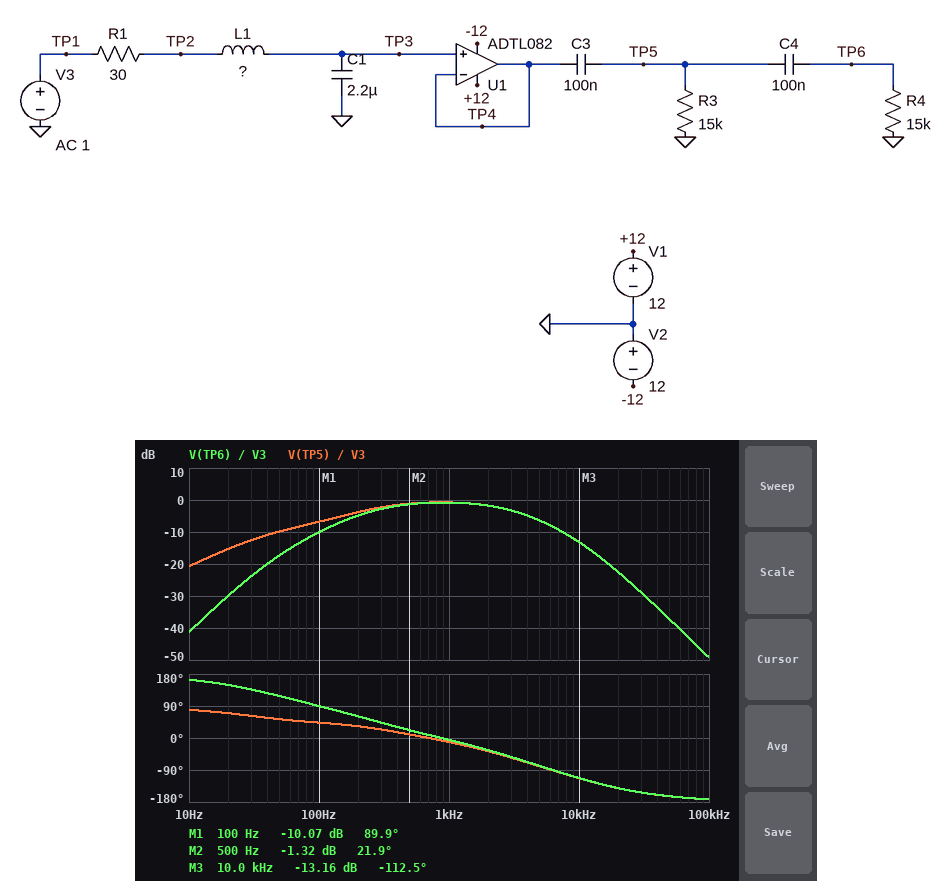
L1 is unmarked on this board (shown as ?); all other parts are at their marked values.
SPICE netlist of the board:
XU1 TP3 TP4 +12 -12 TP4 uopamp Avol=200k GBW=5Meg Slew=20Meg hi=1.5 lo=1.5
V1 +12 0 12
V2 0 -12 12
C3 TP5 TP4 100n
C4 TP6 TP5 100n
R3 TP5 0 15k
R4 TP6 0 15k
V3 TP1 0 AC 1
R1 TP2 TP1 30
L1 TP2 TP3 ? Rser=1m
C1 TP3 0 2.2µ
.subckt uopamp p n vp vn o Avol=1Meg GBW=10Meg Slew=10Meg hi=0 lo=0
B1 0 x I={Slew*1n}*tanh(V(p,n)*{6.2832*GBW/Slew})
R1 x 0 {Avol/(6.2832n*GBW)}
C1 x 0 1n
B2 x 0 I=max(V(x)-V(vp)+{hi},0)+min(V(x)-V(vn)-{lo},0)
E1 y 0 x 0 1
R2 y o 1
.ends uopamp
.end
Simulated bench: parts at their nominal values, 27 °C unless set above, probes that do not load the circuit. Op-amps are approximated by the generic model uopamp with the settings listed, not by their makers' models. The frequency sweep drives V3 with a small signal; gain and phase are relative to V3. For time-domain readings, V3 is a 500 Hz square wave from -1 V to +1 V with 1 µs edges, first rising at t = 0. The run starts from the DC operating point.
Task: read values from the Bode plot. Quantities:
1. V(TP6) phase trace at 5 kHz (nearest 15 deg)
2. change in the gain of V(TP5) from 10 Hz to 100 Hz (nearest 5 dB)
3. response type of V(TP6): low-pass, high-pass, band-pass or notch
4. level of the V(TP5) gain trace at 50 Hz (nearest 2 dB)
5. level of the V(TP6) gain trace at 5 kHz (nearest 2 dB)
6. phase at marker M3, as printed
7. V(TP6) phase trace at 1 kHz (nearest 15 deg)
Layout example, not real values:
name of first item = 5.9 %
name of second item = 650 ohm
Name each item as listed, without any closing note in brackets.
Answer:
V(TP6) phase trace at 5 kHz = -75 deg
change in the gain of V(TP5) from 10 Hz to 100 Hz = 15 dB
response type of V(TP6): low-pass, high-pass, band-pass or notch = band-pass
level of the V(TP5) gain trace at 50 Hz = -10 dB
level of the V(TP6) gain trace at 5 kHz = -6 dB
phase at marker M3, as printed = -112.5 deg
V(TP6) phase trace at 1 kHz = 0 deg
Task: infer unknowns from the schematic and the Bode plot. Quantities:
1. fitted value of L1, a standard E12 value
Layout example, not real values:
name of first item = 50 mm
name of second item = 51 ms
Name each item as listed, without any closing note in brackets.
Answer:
fitted value of L1, a standard E12 value = 330 µH
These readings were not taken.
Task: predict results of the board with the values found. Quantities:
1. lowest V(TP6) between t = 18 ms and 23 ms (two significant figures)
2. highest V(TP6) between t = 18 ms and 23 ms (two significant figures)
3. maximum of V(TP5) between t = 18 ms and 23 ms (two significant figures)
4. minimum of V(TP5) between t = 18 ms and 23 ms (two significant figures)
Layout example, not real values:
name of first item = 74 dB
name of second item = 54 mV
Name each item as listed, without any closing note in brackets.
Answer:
lowest V(TP6) between t = 18 ms and 23 ms = -1.4 V
highest V(TP6) between t = 18 ms and 23 ms = 1.4 V
maximum of V(TP5) between t = 18 ms and 23 ms = 1.2 V
minimum of V(TP5) between t = 18 ms and 23 ms = -1.2 V
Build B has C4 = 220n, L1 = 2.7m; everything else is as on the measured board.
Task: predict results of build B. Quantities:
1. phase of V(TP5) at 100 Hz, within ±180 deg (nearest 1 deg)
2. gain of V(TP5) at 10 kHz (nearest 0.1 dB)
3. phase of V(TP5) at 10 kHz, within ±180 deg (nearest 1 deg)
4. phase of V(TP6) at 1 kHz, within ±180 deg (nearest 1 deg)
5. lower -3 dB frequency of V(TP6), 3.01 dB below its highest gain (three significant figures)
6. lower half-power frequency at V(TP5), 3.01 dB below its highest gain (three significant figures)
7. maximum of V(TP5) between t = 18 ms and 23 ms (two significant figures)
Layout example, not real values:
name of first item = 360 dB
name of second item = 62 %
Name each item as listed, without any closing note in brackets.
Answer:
phase of V(TP5) at 100 Hz, within ±180 deg = 51 deg
gain of V(TP5) at 10 kHz = -27.2 dB
phase of V(TP5) at 10 kHz, within ±180 deg = -168 deg
phase of V(TP6) at 1 kHz, within ±180 deg = -14 deg
lower -3 dB frequency of V(TP6), 3.01 dB below its highest gain = 442 Hz
lower half-power frequency at V(TP5), 3.01 dB below its highest gain = 433 Hz
maximum of V(TP5) between t = 18 ms and 23 ms = 1.7 V
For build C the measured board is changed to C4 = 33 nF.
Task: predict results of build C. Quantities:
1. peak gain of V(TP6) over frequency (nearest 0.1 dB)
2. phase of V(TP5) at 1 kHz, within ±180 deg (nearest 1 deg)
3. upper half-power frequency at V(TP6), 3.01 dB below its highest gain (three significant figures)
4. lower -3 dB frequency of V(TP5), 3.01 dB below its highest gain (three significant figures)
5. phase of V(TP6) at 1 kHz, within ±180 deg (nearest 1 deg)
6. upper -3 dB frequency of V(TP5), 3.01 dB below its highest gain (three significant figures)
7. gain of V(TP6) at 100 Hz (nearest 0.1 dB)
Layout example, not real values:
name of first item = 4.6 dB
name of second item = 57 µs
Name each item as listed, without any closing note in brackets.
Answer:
peak gain of V(TP6) over frequency = -1.3 dB
phase of V(TP5) at 1 kHz, within ±180 deg = -12 deg
upper half-power frequency at V(TP6), 3.01 dB below its highest gain = 3.62 kHz
lower -3 dB frequency of V(TP5), 3.01 dB below its highest gain = 135 Hz
phase of V(TP6) at 1 kHz, within ±180 deg = 6 deg
upper -3 dB frequency of V(TP5), 3.01 dB below its highest gain = 3.40 kHz
gain of V(TP6) at 100 Hz = -15.4 dB
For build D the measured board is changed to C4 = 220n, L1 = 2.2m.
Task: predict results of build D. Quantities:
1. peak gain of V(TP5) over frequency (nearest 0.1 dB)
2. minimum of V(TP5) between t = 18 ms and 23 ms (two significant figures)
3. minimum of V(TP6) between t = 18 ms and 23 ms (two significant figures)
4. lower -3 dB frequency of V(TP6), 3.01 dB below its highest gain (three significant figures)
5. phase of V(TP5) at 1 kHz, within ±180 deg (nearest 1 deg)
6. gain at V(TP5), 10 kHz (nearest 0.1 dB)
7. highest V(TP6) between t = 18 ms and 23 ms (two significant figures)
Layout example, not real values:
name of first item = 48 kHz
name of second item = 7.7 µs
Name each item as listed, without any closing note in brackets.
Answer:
peak gain of V(TP5) over frequency = 1.5 dB
minimum of V(TP5) between t = 18 ms and 23 ms = -1.6 V
minimum of V(TP6) between t = 18 ms and 23 ms = -1.7 V
lower -3 dB frequency of V(TP6), 3.01 dB below its highest gain = 354 Hz
phase of V(TP5) at 1 kHz, within ±180 deg = -15 deg
gain at V(TP5), 10 kHz = -25.4 dB
highest V(TP6) between t = 18 ms and 23 ms = 1.7 V
